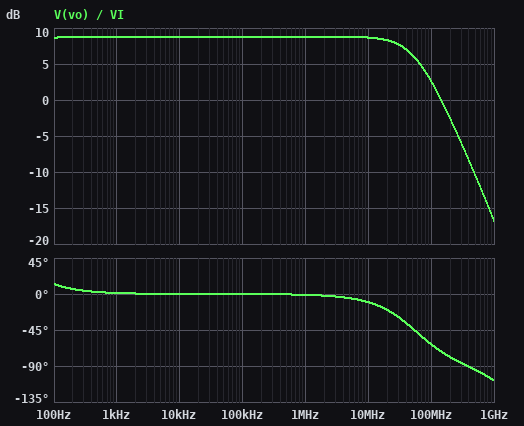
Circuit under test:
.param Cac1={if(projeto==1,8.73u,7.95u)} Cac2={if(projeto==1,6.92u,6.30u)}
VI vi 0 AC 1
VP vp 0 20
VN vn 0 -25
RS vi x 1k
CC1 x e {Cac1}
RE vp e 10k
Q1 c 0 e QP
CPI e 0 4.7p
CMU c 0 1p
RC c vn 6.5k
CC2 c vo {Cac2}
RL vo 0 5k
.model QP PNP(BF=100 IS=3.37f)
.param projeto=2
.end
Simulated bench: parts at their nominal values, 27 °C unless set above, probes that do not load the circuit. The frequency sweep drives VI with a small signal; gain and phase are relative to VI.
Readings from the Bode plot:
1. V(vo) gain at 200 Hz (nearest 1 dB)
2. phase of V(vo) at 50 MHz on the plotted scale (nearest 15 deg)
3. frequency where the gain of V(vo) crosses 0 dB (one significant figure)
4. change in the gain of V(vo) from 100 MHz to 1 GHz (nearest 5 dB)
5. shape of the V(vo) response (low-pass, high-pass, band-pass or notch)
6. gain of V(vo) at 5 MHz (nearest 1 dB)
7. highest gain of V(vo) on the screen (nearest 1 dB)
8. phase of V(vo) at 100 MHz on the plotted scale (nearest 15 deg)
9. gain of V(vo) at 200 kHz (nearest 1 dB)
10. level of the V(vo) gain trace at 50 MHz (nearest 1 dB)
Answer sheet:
9 dB
-45 deg
100 MHz
-20 dB
low-pass
9 dB
9 dB
-60 deg
9 dB
6 dB
